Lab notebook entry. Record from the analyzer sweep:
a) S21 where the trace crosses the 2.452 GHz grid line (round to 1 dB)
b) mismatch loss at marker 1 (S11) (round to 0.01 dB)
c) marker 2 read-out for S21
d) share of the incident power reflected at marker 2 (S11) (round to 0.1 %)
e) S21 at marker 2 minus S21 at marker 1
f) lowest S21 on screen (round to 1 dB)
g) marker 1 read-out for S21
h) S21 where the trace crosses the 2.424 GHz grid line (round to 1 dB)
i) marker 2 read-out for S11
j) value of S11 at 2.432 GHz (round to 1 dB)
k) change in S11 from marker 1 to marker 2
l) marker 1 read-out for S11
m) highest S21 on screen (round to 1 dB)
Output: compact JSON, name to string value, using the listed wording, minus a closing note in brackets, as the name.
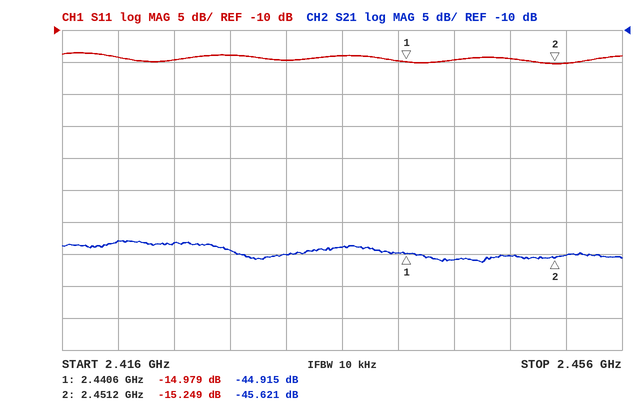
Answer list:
{"S21 where the trace crosses the 2.452 GHz grid line": "-45 dB", "mismatch loss at marker 1 (S11)": "0.14 dB", "marker 2 read-out for S21": "-45.621 dB", "share of the incident power reflected at marker 2 (S11)": "3.0 %", "S21 at marker 2 minus S21 at marker 1": "-0.706 dB", "lowest S21 on screen": "-46 dB", "marker 1 read-out for S21": "-44.915 dB", "S21 where the trace crosses the 2.424 GHz grid line": "-43 dB", "marker 2 read-out for S11": "-15.249 dB", "value of S11 at 2.432 GHz": "-15 dB", "change in S11 from marker 1 to marker 2": "-0.270 dB", "marker 1 read-out for S11": "-14.979 dB", "highest S21 on screen": "-43 dB"}
